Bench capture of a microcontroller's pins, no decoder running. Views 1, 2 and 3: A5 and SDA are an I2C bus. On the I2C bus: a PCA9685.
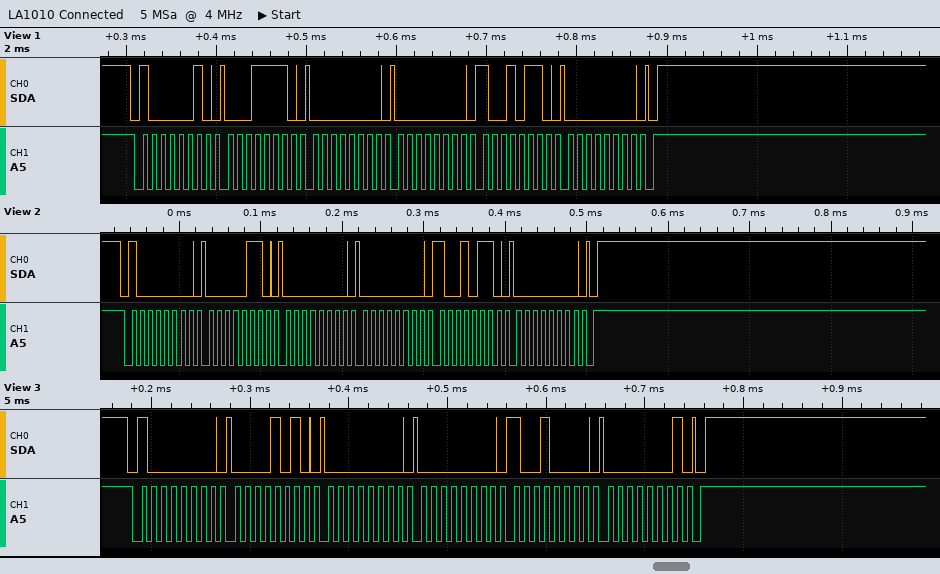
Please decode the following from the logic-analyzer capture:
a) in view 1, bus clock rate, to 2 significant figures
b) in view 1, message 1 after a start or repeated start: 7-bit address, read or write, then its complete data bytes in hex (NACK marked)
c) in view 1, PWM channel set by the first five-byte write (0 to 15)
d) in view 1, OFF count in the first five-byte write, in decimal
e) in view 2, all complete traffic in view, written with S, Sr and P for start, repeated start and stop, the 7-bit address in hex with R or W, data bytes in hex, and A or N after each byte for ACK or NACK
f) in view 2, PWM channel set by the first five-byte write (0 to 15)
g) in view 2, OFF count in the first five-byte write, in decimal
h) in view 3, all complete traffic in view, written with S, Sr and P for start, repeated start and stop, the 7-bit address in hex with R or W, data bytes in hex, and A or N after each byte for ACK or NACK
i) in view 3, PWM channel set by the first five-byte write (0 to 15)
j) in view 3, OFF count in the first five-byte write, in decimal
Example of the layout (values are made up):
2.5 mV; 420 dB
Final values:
100 kHz; 0x41 write: 1E 00 00 96 00; 6; 150; S 40W A 06 A 00 A 00 A 96 A 00 A P; 0; 150; S 40W A 0A A 00 A 00 A 90 A 01 A P; 1; 400
